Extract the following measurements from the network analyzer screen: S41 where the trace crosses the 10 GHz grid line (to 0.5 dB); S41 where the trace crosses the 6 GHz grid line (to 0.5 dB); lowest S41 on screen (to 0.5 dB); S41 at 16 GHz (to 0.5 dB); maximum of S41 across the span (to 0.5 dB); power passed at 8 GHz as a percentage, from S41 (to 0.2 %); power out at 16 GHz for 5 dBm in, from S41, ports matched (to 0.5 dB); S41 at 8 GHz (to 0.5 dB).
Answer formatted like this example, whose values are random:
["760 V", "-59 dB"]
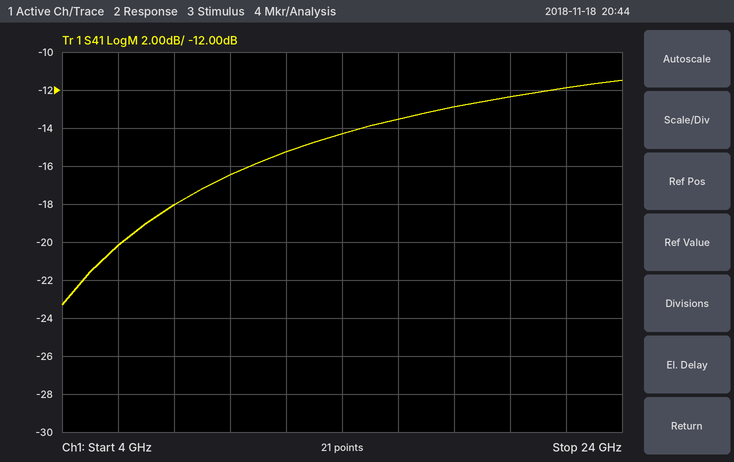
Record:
["-16.5 dB", "-20.0 dB", "-23.5 dB", "-13.5 dB", "-11.5 dB", "1.6 %", "-8.5 dBm", "-18.0 dB"]
